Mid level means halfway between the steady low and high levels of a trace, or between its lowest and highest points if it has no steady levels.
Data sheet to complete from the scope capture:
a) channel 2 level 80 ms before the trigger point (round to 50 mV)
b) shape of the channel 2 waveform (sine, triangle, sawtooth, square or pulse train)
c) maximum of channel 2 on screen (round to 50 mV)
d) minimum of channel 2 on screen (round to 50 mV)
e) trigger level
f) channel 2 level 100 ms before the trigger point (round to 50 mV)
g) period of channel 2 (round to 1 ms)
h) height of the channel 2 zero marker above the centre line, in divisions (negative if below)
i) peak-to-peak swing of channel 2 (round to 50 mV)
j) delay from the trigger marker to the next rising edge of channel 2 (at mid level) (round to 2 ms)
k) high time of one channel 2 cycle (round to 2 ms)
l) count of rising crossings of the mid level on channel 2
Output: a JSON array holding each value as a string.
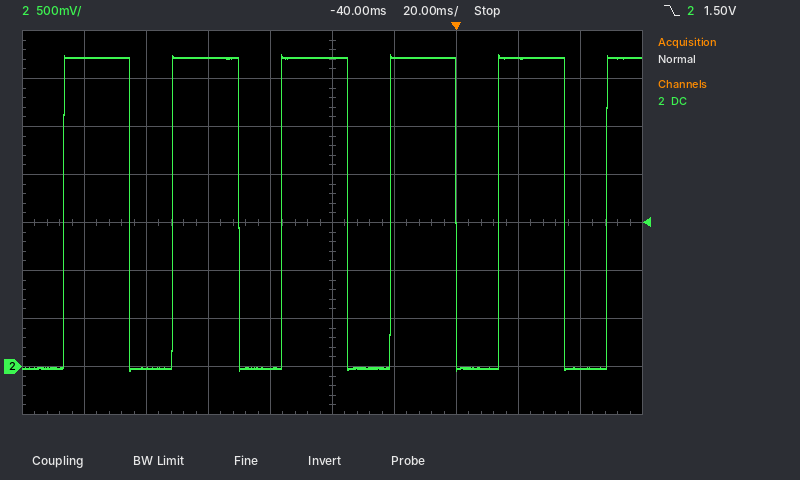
["3.20 V", "pulse train", "3.25 V", "-50 mV", "1.50 V", "0 mV", "35 ms", "-3.0 div", "3.30 V", "14 ms", "22 ms", "6"]
